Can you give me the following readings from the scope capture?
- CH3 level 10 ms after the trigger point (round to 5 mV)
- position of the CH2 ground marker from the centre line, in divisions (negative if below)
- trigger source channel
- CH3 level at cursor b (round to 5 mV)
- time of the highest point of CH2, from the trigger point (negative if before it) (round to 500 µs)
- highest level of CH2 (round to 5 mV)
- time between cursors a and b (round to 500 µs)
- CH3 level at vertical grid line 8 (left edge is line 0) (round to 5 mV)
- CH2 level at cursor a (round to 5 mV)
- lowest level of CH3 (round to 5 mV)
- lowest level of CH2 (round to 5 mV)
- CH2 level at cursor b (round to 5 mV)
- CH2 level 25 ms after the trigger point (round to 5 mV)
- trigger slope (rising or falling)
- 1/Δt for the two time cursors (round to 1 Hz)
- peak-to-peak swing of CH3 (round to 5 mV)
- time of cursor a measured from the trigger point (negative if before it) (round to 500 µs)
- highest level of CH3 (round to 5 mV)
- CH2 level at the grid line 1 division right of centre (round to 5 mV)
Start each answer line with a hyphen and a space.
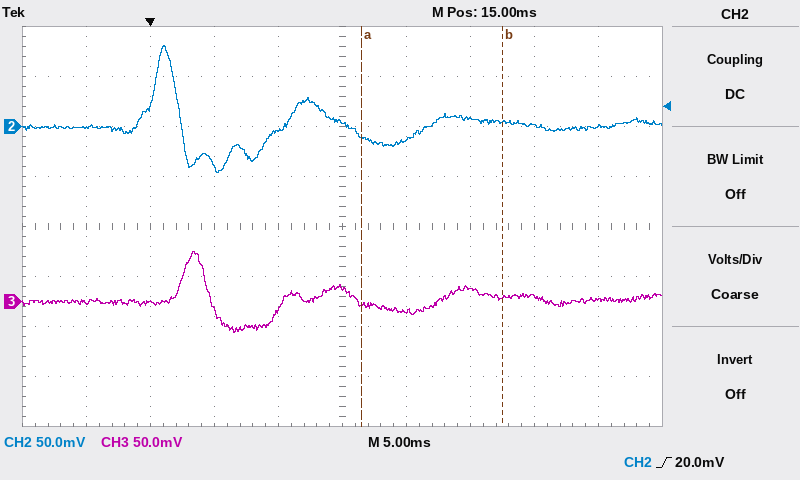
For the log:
- -10 mV
- +2.0 div
- CH2
- 5 mV
- +1.0 ms
- 80 mV
- 11.0 ms
- 5 mV
- -10 mV
- -30 mV
- -45 mV
- 5 mV
- 10 mV
- rising
- 91 Hz
- 80 mV
- +16.5 ms
- 50 mV
- -15 mV
